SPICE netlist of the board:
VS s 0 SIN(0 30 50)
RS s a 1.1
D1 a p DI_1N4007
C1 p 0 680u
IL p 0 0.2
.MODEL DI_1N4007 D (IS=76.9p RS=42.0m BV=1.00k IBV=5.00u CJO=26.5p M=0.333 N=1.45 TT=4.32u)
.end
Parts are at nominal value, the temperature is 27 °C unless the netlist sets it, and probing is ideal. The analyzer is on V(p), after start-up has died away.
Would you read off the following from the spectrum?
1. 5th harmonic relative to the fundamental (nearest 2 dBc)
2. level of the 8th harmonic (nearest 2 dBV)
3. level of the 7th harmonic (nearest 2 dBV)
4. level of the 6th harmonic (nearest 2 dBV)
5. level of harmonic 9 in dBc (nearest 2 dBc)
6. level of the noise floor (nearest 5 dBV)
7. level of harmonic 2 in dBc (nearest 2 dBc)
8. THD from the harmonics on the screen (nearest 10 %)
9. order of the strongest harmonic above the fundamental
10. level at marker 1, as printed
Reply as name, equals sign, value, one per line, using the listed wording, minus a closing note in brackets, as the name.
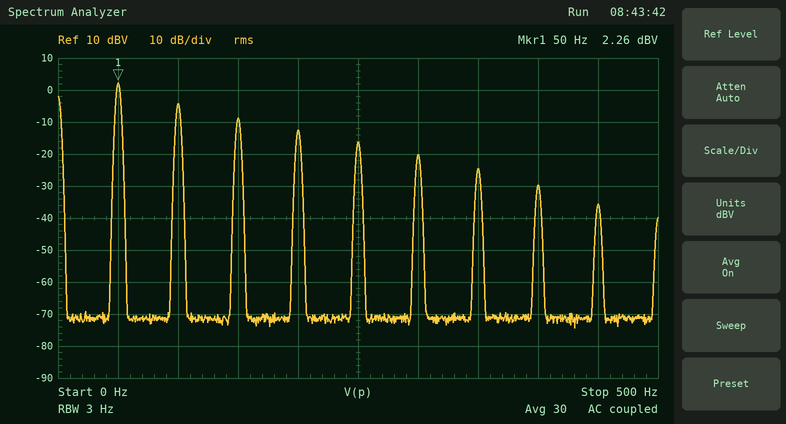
5th harmonic relative to the fundamental = -18 dBc
level of the 8th harmonic = -30 dBV
level of the 7th harmonic = -24 dBV
level of the 6th harmonic = -20 dBV
level of harmonic 9 in dBc = -38 dBc
level of the noise floor = -70 dBV
level of harmonic 2 in dBc = -6 dBc
THD from the harmonics on the screen = 60 %
order of the strongest harmonic above the fundamental = 2
level at marker 1, as printed = 2.26 dBV
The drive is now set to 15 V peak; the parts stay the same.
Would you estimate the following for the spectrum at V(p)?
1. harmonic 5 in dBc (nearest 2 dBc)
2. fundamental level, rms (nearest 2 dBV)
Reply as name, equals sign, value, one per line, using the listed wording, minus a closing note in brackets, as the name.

harmonic 5 in dBc = -22 dBc
fundamental level, rms = 2 dBV
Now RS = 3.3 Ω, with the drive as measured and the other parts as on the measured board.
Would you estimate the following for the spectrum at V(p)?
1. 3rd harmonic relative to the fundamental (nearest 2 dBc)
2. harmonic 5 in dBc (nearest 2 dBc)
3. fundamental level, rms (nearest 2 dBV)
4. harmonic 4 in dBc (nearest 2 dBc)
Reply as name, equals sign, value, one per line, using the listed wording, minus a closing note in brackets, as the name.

3rd harmonic relative to the fundamental = -12 dBc
harmonic 5 in dBc = -24 dBc
fundamental level, rms = 2 dBV
harmonic 4 in dBc = -18 dBc
